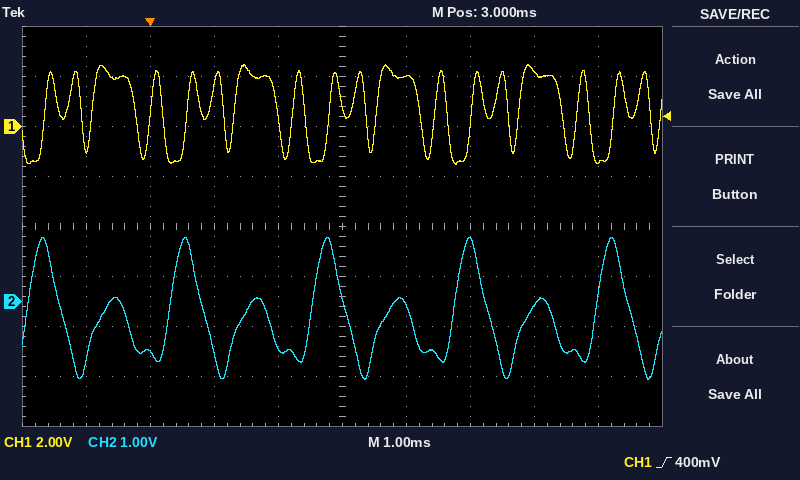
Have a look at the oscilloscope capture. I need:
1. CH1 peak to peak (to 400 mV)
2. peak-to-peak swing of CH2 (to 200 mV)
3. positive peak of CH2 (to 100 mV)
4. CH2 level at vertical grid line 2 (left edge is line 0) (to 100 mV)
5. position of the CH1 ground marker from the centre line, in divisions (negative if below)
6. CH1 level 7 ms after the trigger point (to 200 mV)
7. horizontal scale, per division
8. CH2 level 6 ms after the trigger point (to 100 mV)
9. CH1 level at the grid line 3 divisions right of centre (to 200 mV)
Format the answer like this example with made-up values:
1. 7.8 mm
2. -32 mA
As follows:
1. 4.0 V
2. 2.8 V
3. 1.3 V
4. -1.0 V
5. +2.0 div
6. -1.4 V
7. 1 ms
8. -100 mV
9. 2.2 V
